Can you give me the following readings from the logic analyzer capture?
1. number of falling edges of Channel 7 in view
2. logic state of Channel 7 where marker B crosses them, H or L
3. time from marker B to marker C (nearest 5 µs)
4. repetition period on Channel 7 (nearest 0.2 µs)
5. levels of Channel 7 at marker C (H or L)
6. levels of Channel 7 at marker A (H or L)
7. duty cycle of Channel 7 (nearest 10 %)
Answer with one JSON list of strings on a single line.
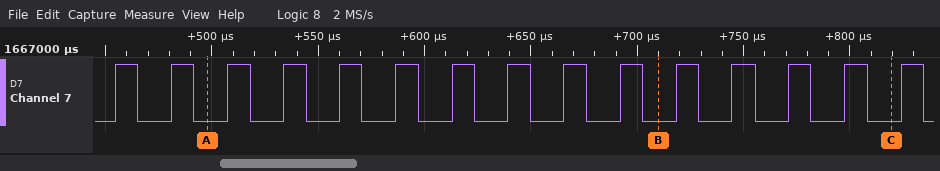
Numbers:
["15", "Channel 7=L", "110 µs", "26.4 µs", "Channel 7=L", "Channel 7=L", "40 %"]
